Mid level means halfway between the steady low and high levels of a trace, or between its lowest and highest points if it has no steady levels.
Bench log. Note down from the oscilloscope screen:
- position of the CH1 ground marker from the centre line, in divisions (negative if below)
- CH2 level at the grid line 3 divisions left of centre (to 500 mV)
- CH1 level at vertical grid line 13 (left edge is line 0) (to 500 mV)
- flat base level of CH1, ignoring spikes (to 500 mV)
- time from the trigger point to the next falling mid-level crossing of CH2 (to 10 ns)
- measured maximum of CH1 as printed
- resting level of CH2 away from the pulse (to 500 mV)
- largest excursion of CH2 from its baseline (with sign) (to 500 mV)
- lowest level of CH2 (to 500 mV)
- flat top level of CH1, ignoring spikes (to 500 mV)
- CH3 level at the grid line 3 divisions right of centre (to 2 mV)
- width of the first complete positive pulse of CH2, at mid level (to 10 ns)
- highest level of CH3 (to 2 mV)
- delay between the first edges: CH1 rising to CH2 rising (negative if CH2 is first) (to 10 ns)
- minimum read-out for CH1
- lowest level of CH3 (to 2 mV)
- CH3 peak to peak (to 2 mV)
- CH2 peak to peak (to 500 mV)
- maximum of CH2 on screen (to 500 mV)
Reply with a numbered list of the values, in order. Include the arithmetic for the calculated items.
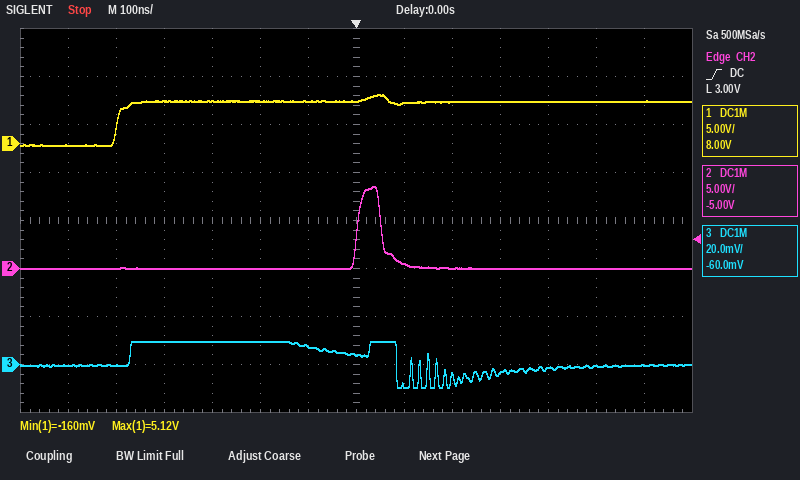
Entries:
1. +1.6 div
2. 0.0 V
3. 4.5 V
4. 0.0 V
5. 50 ns
6. 5.12 V
7. 0.0 V
8. 8.5 V − (0.0 V) = +8.5 V
9. 0.0 V
10. 4.5 V
11. -4 mV
12. 50 ns
13. 10 mV
14. +500 ns
15. -160 mV
16. -10 mV
17. 10 mV − (-10 mV) = 20 mV
18. 8.5 V − (0.0 V) = 8.5 V
19. 8.5 V
